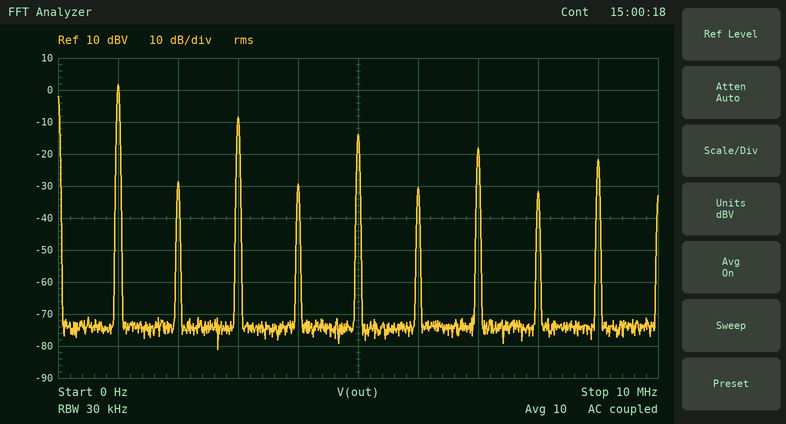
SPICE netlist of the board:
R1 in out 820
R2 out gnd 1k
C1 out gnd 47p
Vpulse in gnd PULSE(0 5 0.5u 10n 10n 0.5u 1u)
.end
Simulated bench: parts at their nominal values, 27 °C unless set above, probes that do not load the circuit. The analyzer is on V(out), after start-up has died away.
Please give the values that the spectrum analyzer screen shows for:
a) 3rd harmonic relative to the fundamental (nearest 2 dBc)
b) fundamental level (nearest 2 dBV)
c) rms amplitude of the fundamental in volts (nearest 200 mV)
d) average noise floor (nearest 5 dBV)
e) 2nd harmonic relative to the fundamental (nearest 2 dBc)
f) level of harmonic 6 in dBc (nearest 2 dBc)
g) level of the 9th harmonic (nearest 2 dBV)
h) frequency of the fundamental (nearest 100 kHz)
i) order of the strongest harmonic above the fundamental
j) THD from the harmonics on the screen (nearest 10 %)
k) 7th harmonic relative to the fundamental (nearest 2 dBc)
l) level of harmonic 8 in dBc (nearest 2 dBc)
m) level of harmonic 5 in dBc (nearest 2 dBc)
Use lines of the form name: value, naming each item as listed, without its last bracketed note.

3rd harmonic relative to the fundamental: -10 dBc
fundamental level: 2 dBV
rms amplitude of the fundamental in volts: 1.2 V
average noise floor: -75 dBV
2nd harmonic relative to the fundamental: -30 dBc
level of harmonic 6 in dBc: -32 dBc
level of the 9th harmonic: -22 dBV
frequency of the fundamental: 1.0 MHz
order of the strongest harmonic above the fundamental: 3
THD from the harmonics on the screen: 40 %
7th harmonic relative to the fundamental: -20 dBc
level of harmonic 8 in dBc: -34 dBc
level of harmonic 5 in dBc: -16 dBc
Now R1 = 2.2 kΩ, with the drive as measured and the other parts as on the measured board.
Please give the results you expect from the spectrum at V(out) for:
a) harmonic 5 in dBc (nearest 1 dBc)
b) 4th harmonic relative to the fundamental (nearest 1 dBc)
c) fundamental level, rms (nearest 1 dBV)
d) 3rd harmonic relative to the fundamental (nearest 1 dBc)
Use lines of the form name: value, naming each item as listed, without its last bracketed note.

harmonic 5 in dBc: -17 dBc
4th harmonic relative to the fundamental: -32 dBc
fundamental level, rms: -3 dBV
3rd harmonic relative to the fundamental: -11 dBc
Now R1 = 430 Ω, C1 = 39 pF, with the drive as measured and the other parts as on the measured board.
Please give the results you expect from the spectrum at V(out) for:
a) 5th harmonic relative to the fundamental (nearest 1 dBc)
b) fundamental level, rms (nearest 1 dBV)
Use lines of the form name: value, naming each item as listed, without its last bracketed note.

5th harmonic relative to the fundamental: -15 dBc
fundamental level, rms: 4 dBV
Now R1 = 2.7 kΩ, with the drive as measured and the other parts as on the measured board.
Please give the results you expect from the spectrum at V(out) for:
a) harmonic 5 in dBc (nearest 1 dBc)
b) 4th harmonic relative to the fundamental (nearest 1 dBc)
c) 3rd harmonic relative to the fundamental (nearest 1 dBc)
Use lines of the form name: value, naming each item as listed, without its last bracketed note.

harmonic 5 in dBc: -17 dBc
4th harmonic relative to the fundamental: -32 dBc
3rd harmonic relative to the fundamental: -11 dBc
